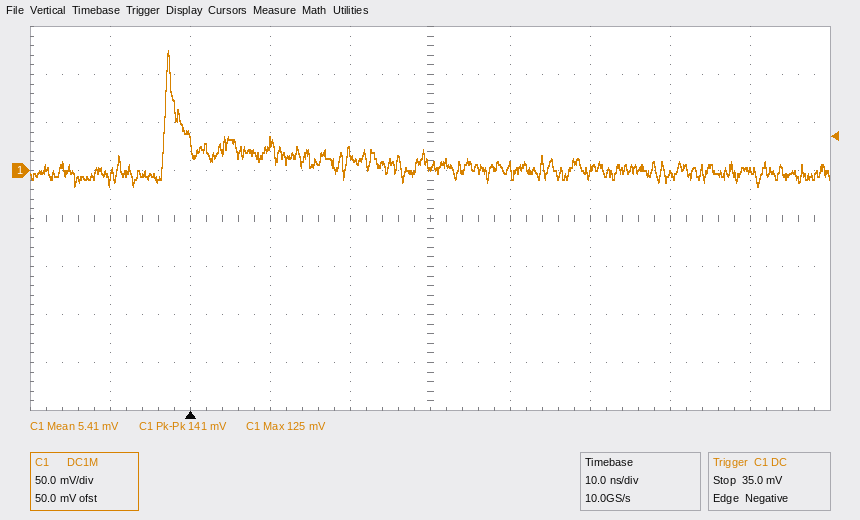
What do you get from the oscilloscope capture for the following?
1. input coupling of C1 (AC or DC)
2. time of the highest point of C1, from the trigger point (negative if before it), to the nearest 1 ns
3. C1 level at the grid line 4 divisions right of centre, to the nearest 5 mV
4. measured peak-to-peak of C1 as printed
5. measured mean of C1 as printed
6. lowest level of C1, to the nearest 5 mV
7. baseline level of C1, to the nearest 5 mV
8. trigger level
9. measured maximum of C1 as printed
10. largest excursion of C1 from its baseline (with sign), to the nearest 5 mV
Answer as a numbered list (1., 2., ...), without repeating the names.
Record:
1. DC
2. -3 ns
3. 0 mV
4. 141 mV
5. 5.41 mV
6. -15 mV
7. 0 mV
8. 35.0 mV
9. 125 mV
10. +125 mV
